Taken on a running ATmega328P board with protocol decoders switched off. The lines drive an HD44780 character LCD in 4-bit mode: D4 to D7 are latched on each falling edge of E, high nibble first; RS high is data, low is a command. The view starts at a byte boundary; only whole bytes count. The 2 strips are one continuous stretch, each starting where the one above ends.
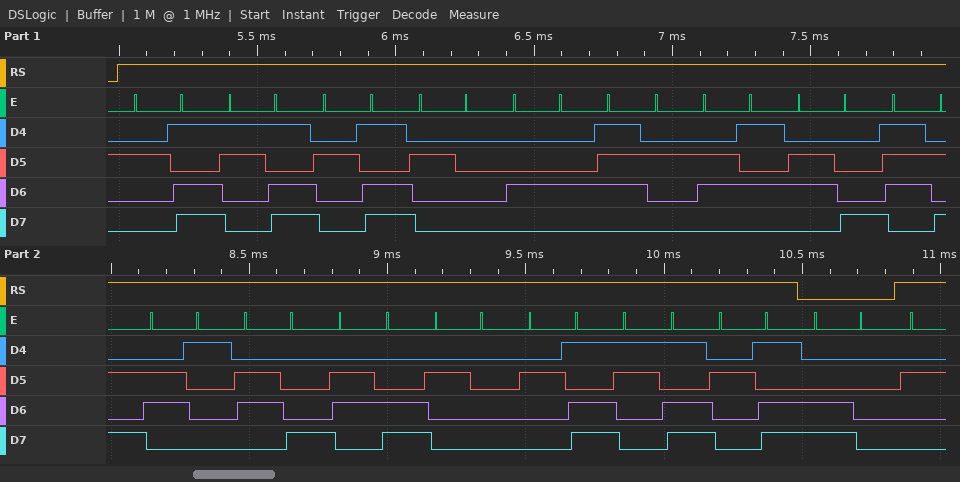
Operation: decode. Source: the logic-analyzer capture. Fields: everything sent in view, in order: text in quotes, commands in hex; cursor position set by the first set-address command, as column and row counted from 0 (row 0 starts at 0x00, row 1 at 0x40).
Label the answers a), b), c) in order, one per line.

a) "-=- Drehzahl -=-" 0xC0
b) column 0, row 1
